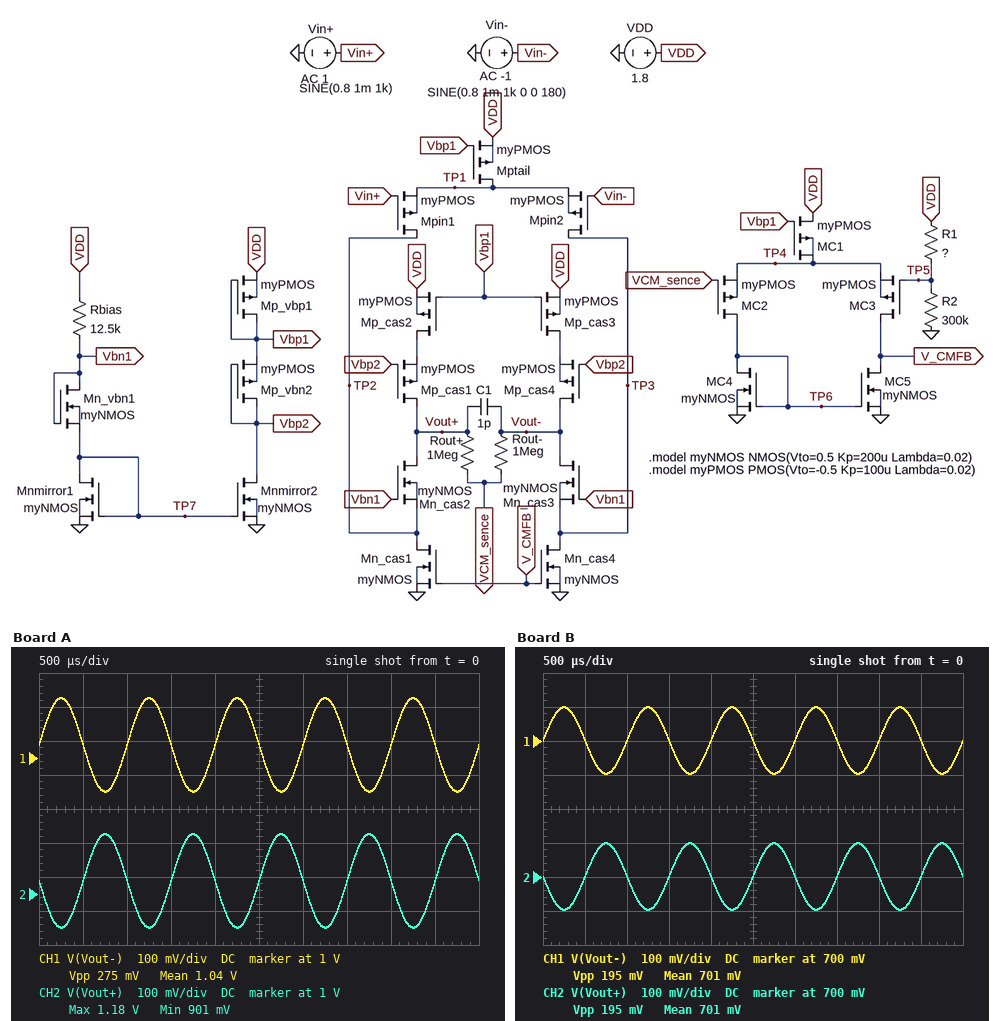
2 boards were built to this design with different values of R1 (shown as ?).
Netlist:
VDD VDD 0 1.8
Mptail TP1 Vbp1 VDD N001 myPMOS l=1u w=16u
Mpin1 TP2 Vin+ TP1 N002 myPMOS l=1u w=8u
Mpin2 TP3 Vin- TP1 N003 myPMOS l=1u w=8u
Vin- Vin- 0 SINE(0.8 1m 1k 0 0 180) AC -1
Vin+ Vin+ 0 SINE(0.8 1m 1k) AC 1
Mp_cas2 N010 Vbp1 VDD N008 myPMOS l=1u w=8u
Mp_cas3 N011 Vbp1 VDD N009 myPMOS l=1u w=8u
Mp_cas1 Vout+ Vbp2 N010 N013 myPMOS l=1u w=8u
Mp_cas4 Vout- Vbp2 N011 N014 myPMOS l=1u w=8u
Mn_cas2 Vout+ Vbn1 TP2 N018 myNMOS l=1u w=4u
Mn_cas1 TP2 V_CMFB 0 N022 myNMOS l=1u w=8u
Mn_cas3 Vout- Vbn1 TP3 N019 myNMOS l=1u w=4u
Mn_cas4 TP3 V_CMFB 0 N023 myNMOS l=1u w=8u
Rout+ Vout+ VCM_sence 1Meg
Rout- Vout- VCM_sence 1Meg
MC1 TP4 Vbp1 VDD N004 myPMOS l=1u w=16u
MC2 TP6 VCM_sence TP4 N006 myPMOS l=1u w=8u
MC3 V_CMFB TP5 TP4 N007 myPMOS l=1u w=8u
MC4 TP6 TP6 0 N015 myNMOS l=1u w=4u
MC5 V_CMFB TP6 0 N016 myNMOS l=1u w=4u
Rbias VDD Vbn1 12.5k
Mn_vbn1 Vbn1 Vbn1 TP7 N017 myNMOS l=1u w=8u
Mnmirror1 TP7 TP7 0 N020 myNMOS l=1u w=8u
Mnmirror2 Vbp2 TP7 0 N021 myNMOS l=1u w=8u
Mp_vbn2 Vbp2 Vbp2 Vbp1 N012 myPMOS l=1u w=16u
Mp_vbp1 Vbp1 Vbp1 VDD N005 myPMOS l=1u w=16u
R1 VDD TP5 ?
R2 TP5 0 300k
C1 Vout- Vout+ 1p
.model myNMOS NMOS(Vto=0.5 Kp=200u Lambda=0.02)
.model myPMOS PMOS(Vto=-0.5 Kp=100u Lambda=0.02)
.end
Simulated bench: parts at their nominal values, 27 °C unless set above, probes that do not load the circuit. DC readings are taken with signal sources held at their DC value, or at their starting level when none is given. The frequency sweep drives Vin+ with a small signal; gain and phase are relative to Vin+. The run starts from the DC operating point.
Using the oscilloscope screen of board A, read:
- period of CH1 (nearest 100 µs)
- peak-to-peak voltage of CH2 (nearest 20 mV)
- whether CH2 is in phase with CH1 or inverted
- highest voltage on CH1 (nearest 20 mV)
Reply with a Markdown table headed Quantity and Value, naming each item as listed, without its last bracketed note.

| Quantity | Value |
|---|---|
| period of CH1 | 1.0 ms |
| peak-to-peak voltage of CH2 | 280 mV |
| whether CH2 is in phase with CH1 or inverted | inverted |
| highest voltage on CH1 | 1.18 V |
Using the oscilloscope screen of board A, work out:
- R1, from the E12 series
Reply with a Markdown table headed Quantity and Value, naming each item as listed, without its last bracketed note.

| Quantity | Value |
|---|---|
| R1, from the E12 series | 220 kΩ |
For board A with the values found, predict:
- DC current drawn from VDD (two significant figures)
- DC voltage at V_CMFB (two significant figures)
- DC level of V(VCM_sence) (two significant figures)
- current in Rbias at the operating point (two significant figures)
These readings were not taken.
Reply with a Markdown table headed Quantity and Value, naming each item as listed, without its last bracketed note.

| Quantity | Value |
|---|---|
| DC current drawn from VDD | 150 µA |
| DC voltage at V_CMFB | 700 mV |
| DC level of V(VCM_sence) | 1.0 V |
| current in Rbias at the operating point | 32 µA |
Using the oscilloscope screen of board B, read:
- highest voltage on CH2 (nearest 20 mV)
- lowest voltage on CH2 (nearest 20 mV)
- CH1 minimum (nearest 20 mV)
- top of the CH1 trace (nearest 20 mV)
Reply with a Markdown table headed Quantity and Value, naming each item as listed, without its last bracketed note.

| Quantity | Value |
|---|---|
| highest voltage on CH2 | 800 mV |
| lowest voltage on CH2 | 600 mV |
| CH1 minimum | 600 mV |
| top of the CH1 trace | 800 mV |
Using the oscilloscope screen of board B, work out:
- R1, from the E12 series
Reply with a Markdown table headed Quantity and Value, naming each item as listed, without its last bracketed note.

| Quantity | Value |
|---|---|
| R1, from the E12 series | 470 kΩ |
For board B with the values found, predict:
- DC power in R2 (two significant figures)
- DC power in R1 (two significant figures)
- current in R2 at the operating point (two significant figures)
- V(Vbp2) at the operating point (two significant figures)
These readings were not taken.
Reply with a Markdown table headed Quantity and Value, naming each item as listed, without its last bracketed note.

| Quantity | Value |
|---|---|
| DC power in R2 | 1.6 µW |
| DC power in R1 | 2.6 µW |
| current in R2 at the operating point | 2.3 µA |
| V(Vbp2) at the operating point | 400 mV |
